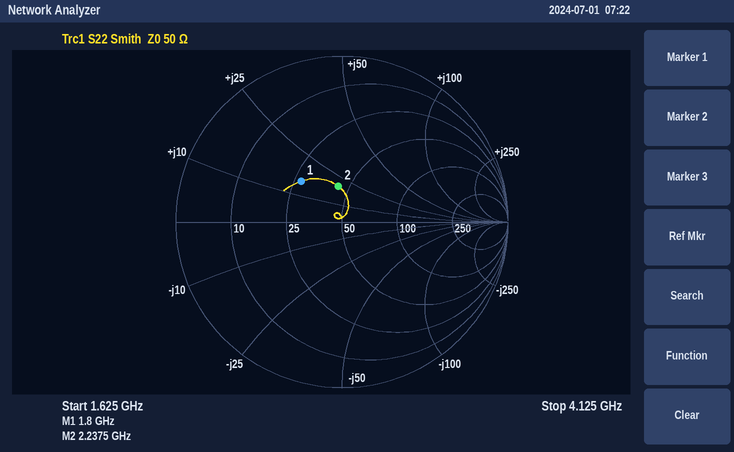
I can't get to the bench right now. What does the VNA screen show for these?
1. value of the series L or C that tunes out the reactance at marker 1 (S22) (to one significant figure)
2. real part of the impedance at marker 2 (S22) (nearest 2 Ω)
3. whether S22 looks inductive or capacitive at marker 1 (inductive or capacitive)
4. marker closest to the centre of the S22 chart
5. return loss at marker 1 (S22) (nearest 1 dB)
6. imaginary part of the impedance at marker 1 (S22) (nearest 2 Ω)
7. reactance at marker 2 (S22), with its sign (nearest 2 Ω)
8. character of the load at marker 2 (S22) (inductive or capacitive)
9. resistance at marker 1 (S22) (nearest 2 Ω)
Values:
6 pF
44 Ω
inductive
marker 2
9 dB
+16 Ω
+20 Ω
inductive
28 Ω
